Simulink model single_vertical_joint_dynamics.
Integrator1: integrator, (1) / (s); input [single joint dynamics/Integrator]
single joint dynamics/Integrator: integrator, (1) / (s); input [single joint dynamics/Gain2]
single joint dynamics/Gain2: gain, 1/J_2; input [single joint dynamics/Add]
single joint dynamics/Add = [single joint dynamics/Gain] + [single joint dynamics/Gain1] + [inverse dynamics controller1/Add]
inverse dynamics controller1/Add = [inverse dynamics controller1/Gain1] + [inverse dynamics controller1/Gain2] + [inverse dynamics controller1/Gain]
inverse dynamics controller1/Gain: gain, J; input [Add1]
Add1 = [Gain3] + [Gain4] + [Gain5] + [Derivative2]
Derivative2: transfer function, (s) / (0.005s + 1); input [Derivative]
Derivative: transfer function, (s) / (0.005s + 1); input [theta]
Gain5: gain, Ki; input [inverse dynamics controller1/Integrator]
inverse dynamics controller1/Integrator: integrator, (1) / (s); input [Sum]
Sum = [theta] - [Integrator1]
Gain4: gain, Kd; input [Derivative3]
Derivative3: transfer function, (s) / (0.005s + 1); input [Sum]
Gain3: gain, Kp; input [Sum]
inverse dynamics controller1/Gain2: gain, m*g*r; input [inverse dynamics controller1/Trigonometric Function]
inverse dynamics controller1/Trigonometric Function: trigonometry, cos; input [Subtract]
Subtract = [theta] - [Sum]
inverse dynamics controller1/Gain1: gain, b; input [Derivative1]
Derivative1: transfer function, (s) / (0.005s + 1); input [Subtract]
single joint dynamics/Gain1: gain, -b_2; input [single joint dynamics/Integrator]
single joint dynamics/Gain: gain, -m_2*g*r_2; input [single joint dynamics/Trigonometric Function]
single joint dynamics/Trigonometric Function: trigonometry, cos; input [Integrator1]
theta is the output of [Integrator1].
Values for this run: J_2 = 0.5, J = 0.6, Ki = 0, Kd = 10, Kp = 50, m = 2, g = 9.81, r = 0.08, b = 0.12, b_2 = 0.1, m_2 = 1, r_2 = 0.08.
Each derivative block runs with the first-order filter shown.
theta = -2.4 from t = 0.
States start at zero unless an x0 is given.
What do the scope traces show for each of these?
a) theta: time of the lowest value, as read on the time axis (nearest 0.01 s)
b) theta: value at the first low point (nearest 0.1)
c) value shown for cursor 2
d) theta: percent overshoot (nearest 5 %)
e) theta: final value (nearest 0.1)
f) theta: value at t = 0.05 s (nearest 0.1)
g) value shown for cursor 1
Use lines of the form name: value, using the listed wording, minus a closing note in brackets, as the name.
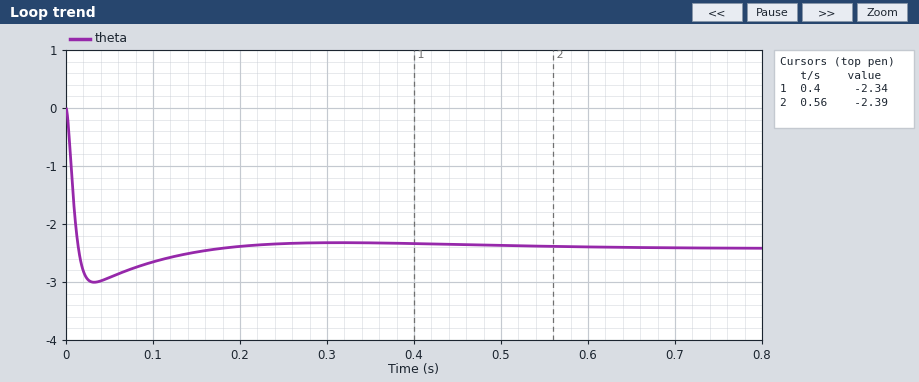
theta: time of the lowest value, as read on the time axis: 0.03 s
theta: value at the first low point: -3.0
value shown for cursor 2: -2.39
theta: percent overshoot: 25 %
theta: final value: -2.4
theta: value at t = 0.05 s: -2.9
value shown for cursor 1: -2.34
